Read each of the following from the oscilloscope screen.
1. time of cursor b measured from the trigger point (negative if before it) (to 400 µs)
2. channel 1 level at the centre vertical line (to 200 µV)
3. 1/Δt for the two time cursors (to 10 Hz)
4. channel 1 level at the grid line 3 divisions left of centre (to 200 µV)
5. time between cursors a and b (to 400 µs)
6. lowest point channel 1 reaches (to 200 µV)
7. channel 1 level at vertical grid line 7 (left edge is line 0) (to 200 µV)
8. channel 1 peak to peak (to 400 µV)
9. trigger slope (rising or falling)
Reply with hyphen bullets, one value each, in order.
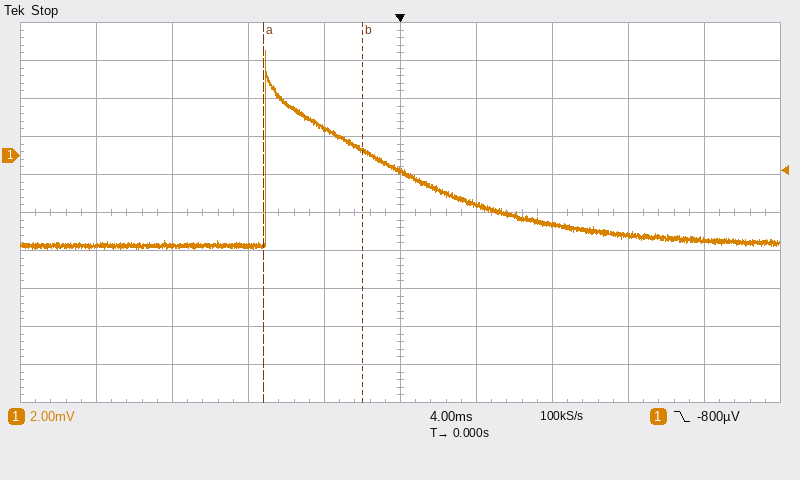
- -2.0 ms
- -800 µV
- 190 Hz
- -4.8 mV
- 5.2 ms
- -5.0 mV
- -3.6 mV
- 10.4 mV
- falling
